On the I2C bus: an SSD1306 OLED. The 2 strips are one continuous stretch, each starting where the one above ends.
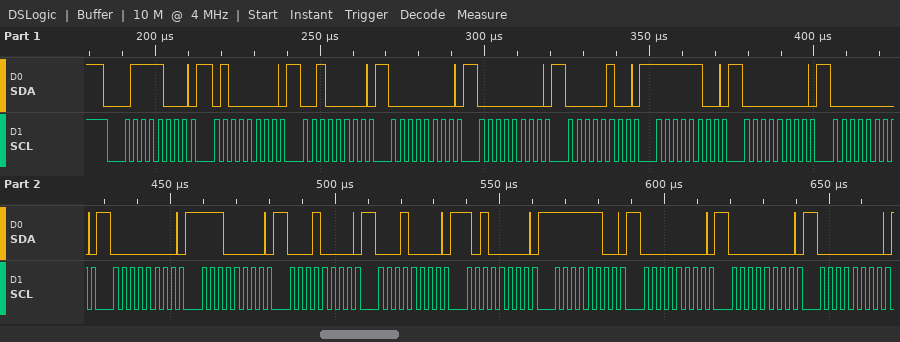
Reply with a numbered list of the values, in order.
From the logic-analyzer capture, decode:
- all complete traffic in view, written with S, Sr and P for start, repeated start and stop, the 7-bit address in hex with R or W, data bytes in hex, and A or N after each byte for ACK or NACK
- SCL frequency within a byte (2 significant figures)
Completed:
1. S 3CW A 40 A 20 A 00 A 00 A 04 A FC A 00 A 00 A 00 A E0 A 10 A 10 A A0 A FC A 00 A 00 A 00 A
2. 400 kHz
